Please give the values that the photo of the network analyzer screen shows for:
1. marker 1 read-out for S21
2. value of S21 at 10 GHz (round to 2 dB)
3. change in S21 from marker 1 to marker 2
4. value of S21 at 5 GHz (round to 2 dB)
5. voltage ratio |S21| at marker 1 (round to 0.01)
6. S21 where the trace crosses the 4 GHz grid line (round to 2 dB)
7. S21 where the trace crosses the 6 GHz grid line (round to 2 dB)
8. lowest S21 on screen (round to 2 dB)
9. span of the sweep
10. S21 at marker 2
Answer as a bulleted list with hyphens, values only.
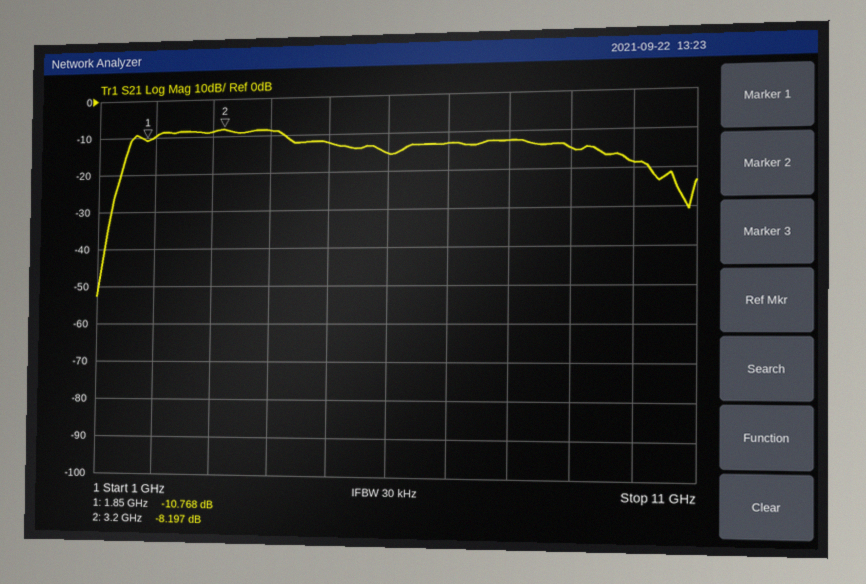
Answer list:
- -10.768 dB
- -18 dB
- 2.571 dB
- -12 dB
- 0.29
- -8 dB
- -16 dB
- -52 dB
- 10 GHz
- -8.197 dB
